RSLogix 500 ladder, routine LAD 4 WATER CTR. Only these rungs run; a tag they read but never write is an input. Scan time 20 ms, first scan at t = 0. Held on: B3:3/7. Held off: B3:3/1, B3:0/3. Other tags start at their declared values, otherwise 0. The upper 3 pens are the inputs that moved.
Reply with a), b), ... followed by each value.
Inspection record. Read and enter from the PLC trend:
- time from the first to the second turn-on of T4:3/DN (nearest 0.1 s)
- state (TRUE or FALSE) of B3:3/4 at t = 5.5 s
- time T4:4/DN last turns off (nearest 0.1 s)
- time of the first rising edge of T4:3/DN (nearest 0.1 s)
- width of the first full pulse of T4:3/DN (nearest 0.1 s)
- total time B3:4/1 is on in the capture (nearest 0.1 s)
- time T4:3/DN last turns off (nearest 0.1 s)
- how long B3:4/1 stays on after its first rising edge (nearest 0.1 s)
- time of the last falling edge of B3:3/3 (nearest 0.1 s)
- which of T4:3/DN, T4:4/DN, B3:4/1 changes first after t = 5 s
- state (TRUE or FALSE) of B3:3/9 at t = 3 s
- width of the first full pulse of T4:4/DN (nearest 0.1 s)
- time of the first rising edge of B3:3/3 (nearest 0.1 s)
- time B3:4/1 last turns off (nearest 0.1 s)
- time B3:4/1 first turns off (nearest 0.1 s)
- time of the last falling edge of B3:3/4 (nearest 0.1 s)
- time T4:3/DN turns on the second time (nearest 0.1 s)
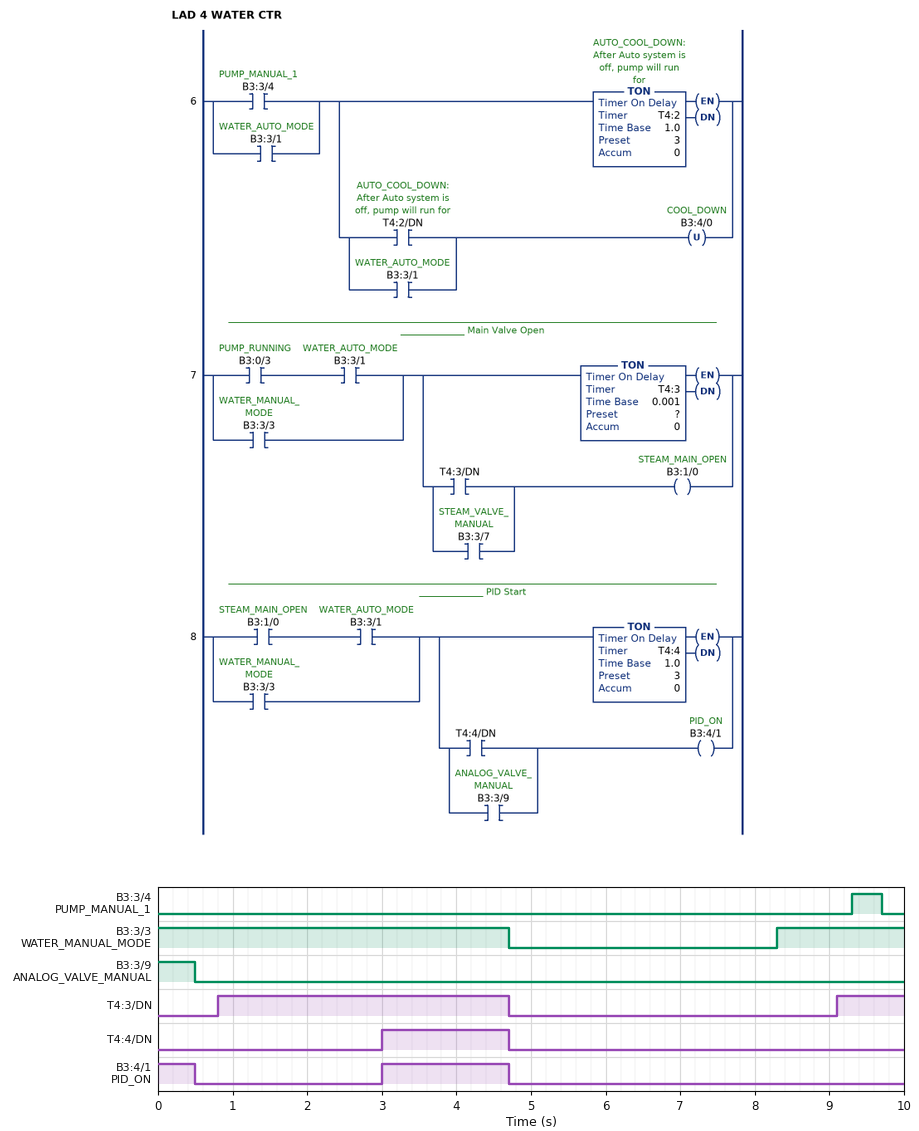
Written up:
a) 8.3 s
b) FALSE
c) 4.7 s
d) 0.8 s
e) 3.9 s
f) 2.2 s
g) 4.7 s
h) 1.7 s
i) 4.7 s
j) T4:3/DN
k) FALSE
l) 1.7 s
m) 8.3 s
n) 4.7 s
o) 0.5 s
p) 9.7 s
q) 9.1 s
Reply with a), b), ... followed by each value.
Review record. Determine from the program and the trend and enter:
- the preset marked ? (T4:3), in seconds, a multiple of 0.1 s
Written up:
a) 0.8 s
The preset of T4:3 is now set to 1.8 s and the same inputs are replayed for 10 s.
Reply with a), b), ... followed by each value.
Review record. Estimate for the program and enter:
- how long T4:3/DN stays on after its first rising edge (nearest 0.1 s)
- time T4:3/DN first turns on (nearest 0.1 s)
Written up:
a) 2.9 s
b) 1.8 s
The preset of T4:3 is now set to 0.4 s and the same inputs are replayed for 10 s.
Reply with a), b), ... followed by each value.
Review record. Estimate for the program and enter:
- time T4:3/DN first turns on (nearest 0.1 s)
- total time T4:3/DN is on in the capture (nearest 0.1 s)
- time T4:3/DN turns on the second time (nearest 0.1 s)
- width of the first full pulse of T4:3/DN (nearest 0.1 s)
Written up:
a) 0.4 s
b) 5.6 s
c) 8.7 s
d) 4.3 s
